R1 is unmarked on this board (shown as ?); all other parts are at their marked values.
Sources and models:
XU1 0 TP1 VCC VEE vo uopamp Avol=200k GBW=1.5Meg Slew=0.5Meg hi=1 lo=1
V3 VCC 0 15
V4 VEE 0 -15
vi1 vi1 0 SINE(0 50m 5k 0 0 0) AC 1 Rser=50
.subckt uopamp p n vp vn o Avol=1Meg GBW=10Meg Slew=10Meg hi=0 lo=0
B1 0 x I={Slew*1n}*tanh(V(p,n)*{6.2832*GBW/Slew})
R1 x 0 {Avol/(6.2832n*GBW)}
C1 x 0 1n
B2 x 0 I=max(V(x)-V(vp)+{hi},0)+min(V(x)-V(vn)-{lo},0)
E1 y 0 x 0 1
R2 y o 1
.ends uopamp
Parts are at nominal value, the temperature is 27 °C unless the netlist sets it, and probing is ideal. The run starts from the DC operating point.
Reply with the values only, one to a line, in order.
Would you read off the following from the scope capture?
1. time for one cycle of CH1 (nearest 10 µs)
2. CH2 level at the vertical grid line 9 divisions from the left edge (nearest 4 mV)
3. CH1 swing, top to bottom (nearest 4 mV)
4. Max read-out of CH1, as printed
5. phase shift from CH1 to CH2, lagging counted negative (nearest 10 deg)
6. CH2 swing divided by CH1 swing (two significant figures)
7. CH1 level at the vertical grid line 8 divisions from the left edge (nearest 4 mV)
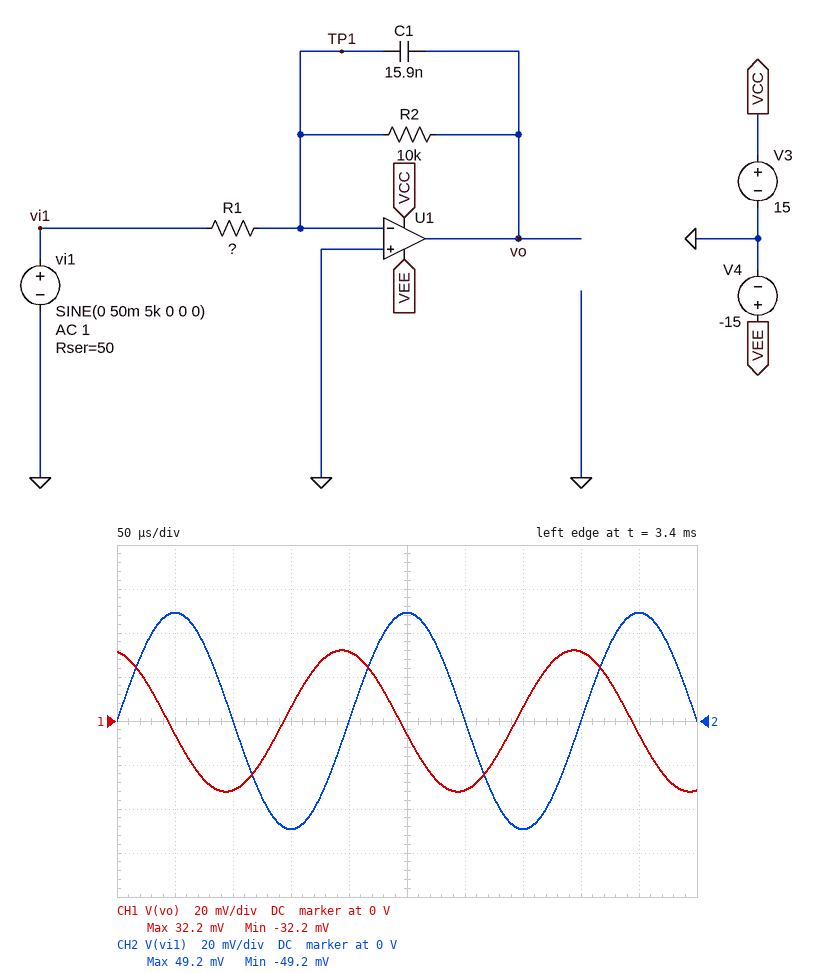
200 µs
48 mV
64 mV
32.2 mV
-100 deg
1.5
32 mV
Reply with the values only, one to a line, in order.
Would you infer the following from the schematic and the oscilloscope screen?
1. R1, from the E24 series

3 kΩ
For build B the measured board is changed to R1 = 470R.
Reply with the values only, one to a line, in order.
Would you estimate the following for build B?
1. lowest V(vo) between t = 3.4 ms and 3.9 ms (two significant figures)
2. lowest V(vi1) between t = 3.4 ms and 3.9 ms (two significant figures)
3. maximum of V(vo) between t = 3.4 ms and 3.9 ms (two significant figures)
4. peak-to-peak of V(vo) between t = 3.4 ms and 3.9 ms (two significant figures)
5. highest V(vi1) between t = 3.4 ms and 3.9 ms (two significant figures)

-190 mV
-45 mV
190 mV
370 mV
45 mV
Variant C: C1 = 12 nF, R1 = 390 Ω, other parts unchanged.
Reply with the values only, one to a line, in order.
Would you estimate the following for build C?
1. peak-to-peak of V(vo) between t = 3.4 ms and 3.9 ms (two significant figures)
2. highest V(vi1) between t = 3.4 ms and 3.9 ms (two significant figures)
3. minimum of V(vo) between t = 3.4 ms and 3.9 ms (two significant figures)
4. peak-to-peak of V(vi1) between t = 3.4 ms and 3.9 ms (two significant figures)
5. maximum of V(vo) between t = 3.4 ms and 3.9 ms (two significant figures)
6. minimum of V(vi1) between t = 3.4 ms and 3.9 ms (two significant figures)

570 mV
44 mV
-290 mV
89 mV
290 mV
-44 mV
